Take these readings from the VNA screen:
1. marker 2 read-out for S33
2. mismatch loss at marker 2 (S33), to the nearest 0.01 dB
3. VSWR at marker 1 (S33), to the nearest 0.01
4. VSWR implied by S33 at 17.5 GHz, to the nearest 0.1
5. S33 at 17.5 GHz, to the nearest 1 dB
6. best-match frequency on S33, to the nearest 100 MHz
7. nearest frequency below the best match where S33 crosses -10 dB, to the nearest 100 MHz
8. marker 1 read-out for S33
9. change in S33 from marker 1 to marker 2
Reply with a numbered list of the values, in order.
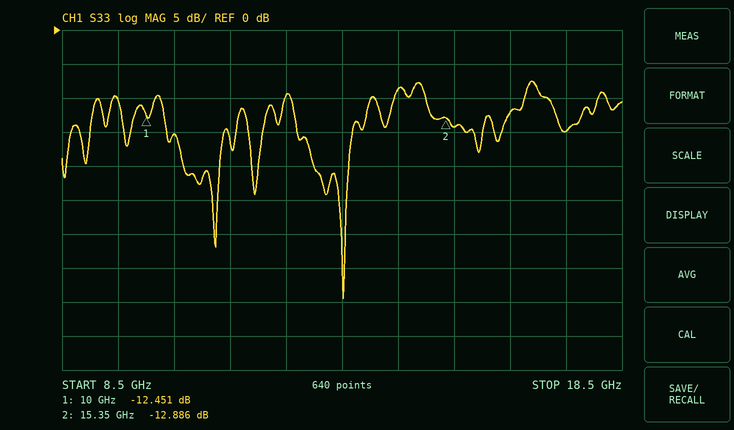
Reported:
1. -12.886 dB
2. 0.23 dB
3. 1.63
4. 1.4
5. -15 dB
6. 13.5 GHz
7. 12.6 GHz
8. -12.451 dB
9. -0.435 dB
